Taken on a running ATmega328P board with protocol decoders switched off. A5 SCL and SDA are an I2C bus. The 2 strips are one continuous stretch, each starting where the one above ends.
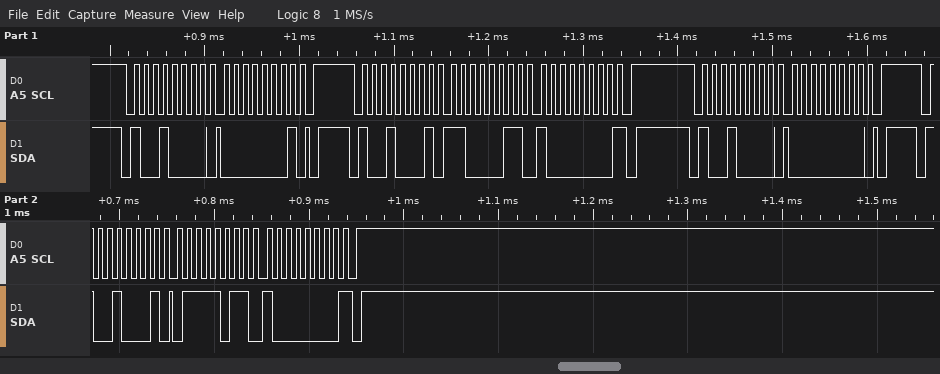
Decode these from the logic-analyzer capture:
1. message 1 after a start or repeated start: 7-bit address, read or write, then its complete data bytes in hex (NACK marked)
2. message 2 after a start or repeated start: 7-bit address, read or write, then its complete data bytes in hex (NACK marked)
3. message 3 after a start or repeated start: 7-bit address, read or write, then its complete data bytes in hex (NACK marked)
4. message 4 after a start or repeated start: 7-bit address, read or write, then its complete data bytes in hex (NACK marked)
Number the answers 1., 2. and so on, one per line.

1. 0x48 write: 01
2. 0x48 read: C3 80 NACK
3. 0x48 write: 00
4. 0x48 read: 7B 80 NACK
